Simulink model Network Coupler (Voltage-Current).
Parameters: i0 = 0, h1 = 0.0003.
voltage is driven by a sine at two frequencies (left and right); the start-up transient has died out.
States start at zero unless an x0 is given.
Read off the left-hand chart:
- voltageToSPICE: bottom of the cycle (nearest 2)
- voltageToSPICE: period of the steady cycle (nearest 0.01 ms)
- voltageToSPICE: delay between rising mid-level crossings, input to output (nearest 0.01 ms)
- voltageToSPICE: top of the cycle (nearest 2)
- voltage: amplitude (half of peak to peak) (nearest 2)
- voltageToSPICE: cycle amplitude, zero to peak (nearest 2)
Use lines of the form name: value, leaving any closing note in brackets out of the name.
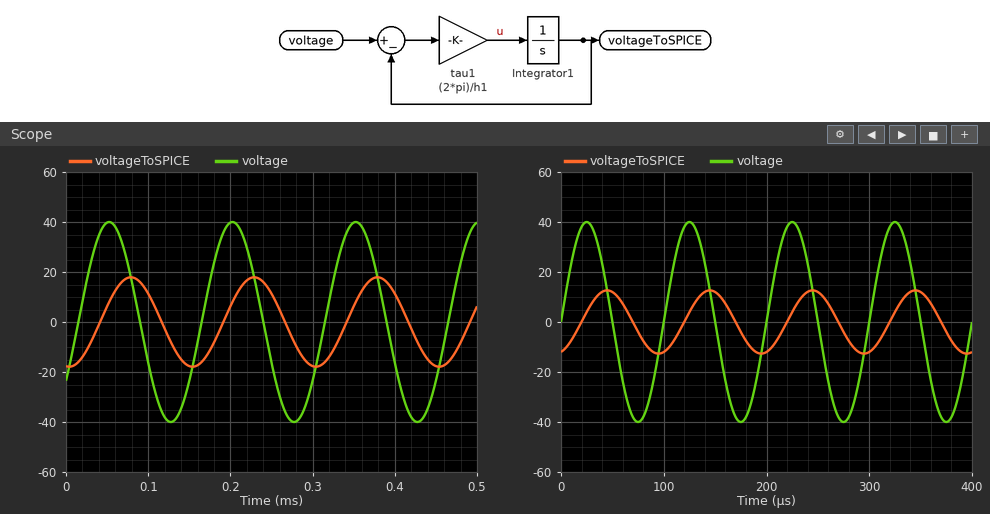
voltageToSPICE: bottom of the cycle: -18
voltageToSPICE: period of the steady cycle: 0.15 ms
voltageToSPICE: delay between rising mid-level crossings, input to output: 0.03 ms
voltageToSPICE: top of the cycle: 18
voltage: amplitude (half of peak to peak): 40
voltageToSPICE: cycle amplitude, zero to peak: 18
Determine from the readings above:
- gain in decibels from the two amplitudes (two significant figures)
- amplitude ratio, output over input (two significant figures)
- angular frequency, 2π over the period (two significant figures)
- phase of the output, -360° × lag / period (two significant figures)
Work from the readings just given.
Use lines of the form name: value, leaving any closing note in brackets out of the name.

gain in decibels from the two amplitudes: -6.9 dB
amplitude ratio, output over input: 0.45
angular frequency, 2π over the period: 42 rad/ms
phase of the output, -360° × lag / period: -72°
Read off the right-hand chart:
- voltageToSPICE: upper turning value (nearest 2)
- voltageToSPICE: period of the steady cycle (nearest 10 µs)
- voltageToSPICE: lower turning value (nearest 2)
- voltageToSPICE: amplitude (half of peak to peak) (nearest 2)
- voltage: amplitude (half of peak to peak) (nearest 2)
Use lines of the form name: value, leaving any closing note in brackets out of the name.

voltageToSPICE: upper turning value: 12
voltageToSPICE: period of the steady cycle: 100 µs
voltageToSPICE: lower turning value: -12
voltageToSPICE: amplitude (half of peak to peak): 12
voltage: amplitude (half of peak to peak): 40
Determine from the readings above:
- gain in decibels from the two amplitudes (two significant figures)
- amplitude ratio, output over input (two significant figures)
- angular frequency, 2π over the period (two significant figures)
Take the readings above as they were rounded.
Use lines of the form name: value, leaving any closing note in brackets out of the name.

gain in decibels from the two amplitudes: -10 dB
amplitude ratio, output over input: 0.30
angular frequency, 2π over the period: 0.063 rad/µs
